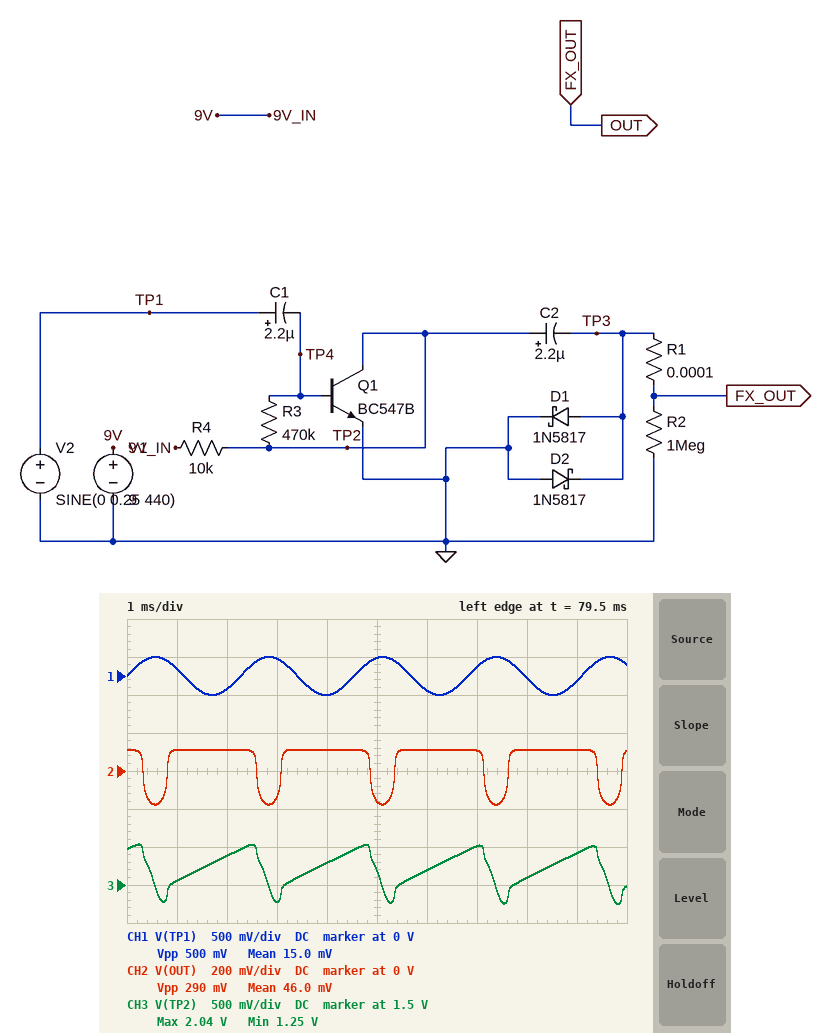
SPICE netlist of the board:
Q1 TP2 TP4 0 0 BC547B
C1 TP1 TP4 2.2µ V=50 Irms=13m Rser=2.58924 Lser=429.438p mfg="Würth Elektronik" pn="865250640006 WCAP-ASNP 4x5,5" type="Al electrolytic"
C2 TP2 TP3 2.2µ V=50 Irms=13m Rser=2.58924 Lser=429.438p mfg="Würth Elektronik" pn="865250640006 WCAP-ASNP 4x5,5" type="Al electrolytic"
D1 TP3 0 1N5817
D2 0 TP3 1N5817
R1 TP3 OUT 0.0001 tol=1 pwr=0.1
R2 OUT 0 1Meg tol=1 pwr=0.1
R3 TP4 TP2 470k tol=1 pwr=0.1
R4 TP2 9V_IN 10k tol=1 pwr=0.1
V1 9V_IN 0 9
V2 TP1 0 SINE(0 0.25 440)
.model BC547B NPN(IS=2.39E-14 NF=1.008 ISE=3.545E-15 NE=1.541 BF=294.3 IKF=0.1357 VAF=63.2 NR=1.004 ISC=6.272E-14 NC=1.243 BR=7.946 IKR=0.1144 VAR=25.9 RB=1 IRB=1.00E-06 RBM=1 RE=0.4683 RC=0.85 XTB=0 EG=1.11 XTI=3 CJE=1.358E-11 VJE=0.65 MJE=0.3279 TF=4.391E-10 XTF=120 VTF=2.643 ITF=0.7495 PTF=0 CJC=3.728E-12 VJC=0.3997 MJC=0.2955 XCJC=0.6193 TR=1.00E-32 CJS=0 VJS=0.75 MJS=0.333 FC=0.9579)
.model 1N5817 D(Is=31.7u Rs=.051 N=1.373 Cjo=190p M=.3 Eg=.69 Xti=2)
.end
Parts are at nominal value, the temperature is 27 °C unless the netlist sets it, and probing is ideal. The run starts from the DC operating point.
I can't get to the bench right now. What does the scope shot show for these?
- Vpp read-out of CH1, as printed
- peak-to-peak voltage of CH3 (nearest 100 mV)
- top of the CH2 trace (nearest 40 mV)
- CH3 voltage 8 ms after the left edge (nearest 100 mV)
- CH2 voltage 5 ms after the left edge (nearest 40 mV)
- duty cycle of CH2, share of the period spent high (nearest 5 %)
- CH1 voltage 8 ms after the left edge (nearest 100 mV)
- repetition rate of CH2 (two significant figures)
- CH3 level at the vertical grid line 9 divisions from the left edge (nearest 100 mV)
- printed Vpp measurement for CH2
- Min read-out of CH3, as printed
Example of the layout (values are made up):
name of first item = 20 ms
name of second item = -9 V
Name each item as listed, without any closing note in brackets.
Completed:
Vpp read-out of CH1, as printed = 500 mV
peak-to-peak voltage of CH3 = 800 mV
top of the CH2 trace = 120 mV
CH3 voltage 8 ms after the left edge = 1.6 V
CH2 voltage 5 ms after the left edge = -160 mV
duty cycle of CH2, share of the period spent high = 80 %
CH1 voltage 8 ms after the left edge = 0 V
repetition rate of CH2 = 440 Hz
CH3 level at the vertical grid line 9 divisions from the left edge = 1.9 V
printed Vpp measurement for CH2 = 290 mV
Min read-out of CH3, as printed = 1.25 V
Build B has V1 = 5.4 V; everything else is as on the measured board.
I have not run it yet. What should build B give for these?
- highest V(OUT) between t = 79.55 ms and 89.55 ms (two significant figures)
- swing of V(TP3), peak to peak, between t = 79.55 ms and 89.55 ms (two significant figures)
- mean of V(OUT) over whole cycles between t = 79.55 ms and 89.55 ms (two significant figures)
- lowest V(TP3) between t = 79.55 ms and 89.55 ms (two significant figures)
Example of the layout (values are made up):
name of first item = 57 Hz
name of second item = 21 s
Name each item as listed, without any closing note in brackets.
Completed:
highest V(OUT) between t = 79.55 ms and 89.55 ms = 93 mV
swing of V(TP3), peak to peak, between t = 79.55 ms and 89.55 ms = 250 mV
mean of V(OUT) over whole cycles between t = 79.55 ms and 89.55 ms = 44 mV
lowest V(TP3) between t = 79.55 ms and 89.55 ms = -160 mV
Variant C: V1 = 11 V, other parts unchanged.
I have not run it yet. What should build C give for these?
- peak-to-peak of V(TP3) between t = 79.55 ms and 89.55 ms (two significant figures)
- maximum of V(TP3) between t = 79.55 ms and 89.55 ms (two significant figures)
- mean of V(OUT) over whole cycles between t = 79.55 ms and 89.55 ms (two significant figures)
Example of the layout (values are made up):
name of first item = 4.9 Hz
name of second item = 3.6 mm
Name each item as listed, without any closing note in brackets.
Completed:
peak-to-peak of V(TP3) between t = 79.55 ms and 89.55 ms = 300 mV
maximum of V(TP3) between t = 79.55 ms and 89.55 ms = 120 mV
mean of V(OUT) over whole cycles between t = 79.55 ms and 89.55 ms = 58 mV
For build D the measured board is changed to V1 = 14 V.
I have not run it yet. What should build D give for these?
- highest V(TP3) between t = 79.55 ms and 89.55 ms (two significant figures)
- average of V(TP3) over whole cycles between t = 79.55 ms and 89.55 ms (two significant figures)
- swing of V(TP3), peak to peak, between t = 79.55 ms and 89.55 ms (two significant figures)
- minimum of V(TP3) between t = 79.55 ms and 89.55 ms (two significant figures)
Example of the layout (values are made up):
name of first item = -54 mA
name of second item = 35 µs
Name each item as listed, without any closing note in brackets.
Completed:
highest V(TP3) between t = 79.55 ms and 89.55 ms = 130 mV
average of V(TP3) over whole cycles between t = 79.55 ms and 89.55 ms = 63 mV
swing of V(TP3), peak to peak, between t = 79.55 ms and 89.55 ms = 320 mV
minimum of V(TP3) between t = 79.55 ms and 89.55 ms = -190 mV
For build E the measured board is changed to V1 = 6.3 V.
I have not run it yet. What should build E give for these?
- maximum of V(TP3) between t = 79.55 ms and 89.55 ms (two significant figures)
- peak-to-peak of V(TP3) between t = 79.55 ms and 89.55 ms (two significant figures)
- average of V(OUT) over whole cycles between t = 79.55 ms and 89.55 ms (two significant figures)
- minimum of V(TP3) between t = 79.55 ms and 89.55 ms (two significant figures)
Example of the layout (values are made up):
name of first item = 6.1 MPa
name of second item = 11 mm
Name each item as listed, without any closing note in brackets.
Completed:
maximum of V(TP3) between t = 79.55 ms and 89.55 ms = 99 mV
peak-to-peak of V(TP3) between t = 79.55 ms and 89.55 ms = 260 mV
average of V(OUT) over whole cycles between t = 79.55 ms and 89.55 ms = 47 mV
minimum of V(TP3) between t = 79.55 ms and 89.55 ms = -160 mV
